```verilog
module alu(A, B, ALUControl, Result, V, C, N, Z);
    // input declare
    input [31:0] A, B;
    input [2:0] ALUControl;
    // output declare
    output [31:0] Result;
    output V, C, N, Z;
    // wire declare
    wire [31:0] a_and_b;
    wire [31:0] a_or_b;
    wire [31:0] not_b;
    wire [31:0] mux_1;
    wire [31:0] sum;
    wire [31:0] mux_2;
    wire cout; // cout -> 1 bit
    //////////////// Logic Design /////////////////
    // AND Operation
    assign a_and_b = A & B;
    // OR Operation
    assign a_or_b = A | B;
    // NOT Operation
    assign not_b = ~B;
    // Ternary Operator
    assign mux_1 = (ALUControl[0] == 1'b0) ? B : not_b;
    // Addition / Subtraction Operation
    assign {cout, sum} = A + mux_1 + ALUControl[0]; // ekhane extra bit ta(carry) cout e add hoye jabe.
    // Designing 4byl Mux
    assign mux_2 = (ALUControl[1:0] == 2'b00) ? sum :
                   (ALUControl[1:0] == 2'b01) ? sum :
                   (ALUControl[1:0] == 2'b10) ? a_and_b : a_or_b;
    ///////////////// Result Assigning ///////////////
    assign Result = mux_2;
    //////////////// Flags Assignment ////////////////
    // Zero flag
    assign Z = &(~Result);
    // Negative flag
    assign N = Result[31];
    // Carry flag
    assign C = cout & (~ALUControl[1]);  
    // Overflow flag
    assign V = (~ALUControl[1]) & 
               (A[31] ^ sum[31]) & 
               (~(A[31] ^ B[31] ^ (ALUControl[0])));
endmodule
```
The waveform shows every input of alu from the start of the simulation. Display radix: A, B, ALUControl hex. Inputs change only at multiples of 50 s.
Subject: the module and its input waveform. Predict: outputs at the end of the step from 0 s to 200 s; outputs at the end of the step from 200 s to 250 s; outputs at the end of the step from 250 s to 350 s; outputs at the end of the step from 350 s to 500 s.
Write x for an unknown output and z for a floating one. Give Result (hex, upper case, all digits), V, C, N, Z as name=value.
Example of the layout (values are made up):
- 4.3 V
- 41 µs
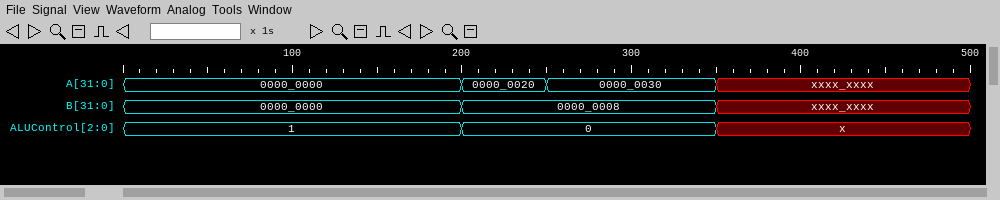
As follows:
- Result=00000000, V=0, C=1, N=0, Z=1
- Result=00000028, V=0, C=0, N=0, Z=0
- Result=00000038, V=0, C=0, N=0, Z=0
- Result=x, V=x, C=x, N=x, Z=x
